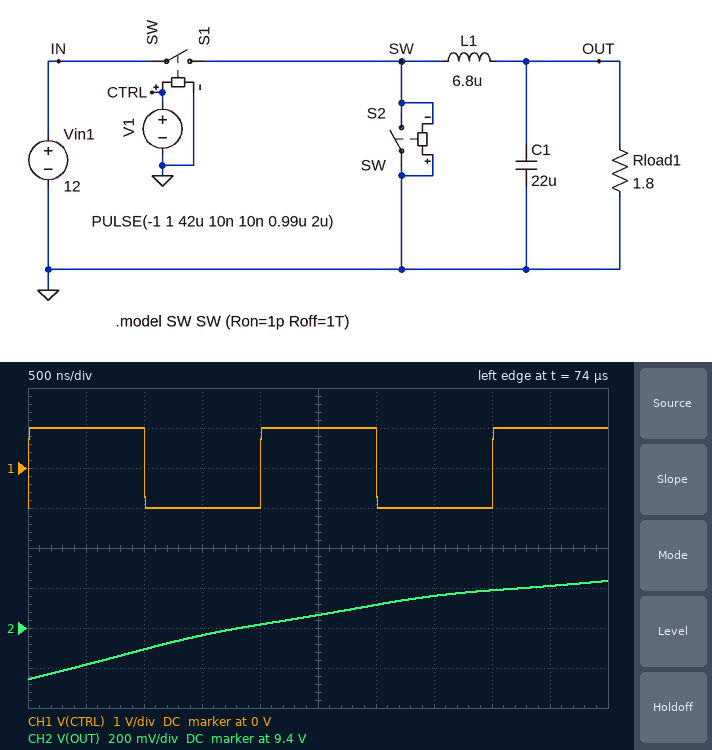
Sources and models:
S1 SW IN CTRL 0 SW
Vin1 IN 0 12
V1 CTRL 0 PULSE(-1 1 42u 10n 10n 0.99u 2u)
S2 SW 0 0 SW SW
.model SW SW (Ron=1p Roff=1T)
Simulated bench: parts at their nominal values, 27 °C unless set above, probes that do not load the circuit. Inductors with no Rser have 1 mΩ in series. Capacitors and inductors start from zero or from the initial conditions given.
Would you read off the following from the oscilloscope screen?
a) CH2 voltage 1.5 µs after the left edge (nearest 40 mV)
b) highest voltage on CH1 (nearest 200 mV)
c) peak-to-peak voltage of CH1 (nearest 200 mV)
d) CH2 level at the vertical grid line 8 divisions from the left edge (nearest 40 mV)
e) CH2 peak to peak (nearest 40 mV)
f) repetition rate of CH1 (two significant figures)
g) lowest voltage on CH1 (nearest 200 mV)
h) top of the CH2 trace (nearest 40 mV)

9.36 V
1.0 V
2.0 V
9.60 V
480 mV
500 kHz
-1.0 V
9.64 V
